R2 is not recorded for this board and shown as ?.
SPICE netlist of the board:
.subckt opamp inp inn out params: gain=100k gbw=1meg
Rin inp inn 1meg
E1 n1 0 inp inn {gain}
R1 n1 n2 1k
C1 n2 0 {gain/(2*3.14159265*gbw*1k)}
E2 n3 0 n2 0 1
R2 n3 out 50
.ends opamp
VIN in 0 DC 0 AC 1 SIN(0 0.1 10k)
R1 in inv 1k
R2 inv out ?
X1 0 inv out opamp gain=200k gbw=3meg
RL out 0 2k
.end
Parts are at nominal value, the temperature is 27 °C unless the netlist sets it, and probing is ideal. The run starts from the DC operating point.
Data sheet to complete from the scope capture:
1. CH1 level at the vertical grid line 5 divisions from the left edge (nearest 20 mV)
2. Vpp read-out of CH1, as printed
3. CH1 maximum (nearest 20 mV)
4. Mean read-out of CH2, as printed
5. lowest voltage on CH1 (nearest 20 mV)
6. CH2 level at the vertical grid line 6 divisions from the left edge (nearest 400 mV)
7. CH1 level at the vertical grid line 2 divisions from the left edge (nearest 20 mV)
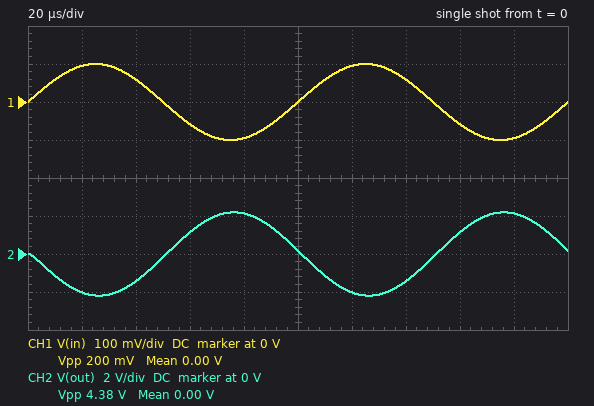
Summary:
0 V
200 mV
100 mV
0.00 V
-100 mV
-2.0 V
60 mV
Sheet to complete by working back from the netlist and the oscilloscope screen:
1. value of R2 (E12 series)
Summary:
22 kΩ
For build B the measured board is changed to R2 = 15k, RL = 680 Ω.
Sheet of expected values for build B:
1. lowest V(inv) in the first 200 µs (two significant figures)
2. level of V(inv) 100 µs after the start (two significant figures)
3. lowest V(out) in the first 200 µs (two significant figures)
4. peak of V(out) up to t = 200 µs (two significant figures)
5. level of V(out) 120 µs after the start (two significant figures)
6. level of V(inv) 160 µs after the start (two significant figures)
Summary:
-5.4 mV
5.4 mV
-1.5 V
1.5 V
-1.4 V
-4.5 mV
